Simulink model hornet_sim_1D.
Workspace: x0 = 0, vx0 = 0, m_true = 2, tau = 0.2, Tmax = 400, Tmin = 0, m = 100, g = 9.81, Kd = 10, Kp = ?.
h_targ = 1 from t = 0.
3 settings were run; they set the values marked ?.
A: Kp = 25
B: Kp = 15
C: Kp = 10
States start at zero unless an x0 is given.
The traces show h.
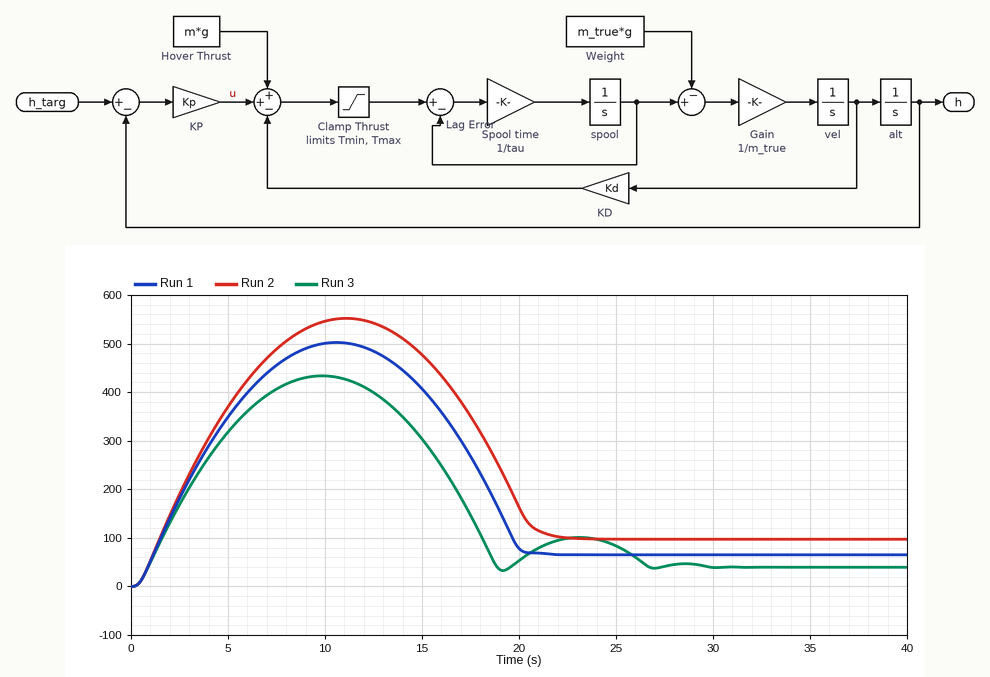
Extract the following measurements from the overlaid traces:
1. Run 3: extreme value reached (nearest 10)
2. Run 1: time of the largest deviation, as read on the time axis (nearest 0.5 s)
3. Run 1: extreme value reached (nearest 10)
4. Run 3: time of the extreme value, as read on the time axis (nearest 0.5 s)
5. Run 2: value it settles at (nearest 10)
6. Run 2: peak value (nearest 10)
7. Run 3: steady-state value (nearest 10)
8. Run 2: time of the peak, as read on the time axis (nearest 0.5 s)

430
10.5 s
500
10.0 s
100
550
40
11.0 s
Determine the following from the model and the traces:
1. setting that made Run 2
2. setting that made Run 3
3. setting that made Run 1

C
A
B
